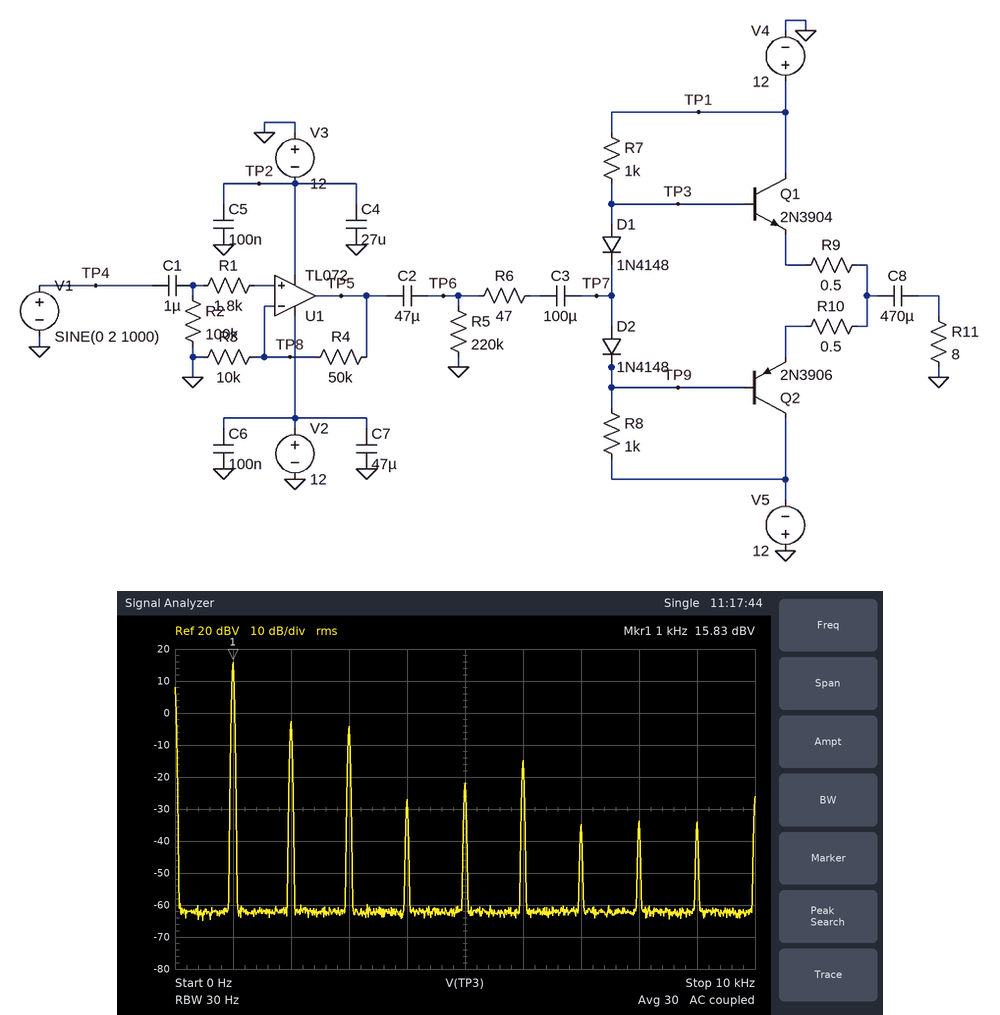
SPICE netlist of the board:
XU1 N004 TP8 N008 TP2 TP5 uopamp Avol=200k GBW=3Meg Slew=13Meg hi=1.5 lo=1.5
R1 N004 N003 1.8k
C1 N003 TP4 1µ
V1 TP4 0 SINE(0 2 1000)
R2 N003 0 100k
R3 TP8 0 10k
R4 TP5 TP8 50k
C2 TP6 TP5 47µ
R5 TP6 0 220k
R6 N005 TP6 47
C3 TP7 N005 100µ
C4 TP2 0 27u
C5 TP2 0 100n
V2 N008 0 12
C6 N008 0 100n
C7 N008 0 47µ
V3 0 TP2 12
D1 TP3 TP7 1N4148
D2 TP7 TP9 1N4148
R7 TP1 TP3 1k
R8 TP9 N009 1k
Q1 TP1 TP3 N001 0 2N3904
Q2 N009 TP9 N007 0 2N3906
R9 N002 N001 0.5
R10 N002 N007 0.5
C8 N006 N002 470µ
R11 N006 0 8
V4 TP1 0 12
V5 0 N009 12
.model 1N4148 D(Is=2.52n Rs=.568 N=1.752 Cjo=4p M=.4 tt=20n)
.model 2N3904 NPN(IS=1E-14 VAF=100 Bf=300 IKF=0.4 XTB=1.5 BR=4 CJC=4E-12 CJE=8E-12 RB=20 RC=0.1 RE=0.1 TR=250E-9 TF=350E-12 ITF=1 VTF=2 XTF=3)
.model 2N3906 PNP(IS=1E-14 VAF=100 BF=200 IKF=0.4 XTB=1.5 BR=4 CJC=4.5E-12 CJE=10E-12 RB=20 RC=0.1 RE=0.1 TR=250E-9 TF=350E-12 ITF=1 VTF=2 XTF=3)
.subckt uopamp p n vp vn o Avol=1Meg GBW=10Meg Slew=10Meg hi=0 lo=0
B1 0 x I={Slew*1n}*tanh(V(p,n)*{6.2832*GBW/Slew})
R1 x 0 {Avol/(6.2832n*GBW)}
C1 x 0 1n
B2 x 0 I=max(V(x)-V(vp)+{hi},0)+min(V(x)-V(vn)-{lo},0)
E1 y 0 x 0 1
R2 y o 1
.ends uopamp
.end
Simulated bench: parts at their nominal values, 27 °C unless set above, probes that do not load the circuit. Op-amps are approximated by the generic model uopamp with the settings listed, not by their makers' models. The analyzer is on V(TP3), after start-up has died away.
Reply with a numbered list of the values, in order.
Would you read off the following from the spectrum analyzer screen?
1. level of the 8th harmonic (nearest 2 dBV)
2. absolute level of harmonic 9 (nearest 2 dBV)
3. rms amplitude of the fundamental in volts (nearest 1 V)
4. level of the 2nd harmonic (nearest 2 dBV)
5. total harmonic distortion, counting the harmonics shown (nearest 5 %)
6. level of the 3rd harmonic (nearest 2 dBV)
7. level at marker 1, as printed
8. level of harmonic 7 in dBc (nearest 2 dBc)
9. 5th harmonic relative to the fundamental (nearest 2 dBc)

1. -34 dBV
2. -34 dBV
3. 6 V
4. -2 dBV
5. 15 %
6. -4 dBV
7. 15.83 dBV
8. -50 dBc
9. -38 dBc
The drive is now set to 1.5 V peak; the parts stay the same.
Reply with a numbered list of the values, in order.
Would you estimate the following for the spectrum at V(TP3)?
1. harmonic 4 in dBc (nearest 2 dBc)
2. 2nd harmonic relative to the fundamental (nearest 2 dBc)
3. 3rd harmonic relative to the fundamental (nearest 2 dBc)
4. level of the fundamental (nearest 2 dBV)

1. -30 dBc
2. -24 dBc
3. -28 dBc
4. 14 dBV
